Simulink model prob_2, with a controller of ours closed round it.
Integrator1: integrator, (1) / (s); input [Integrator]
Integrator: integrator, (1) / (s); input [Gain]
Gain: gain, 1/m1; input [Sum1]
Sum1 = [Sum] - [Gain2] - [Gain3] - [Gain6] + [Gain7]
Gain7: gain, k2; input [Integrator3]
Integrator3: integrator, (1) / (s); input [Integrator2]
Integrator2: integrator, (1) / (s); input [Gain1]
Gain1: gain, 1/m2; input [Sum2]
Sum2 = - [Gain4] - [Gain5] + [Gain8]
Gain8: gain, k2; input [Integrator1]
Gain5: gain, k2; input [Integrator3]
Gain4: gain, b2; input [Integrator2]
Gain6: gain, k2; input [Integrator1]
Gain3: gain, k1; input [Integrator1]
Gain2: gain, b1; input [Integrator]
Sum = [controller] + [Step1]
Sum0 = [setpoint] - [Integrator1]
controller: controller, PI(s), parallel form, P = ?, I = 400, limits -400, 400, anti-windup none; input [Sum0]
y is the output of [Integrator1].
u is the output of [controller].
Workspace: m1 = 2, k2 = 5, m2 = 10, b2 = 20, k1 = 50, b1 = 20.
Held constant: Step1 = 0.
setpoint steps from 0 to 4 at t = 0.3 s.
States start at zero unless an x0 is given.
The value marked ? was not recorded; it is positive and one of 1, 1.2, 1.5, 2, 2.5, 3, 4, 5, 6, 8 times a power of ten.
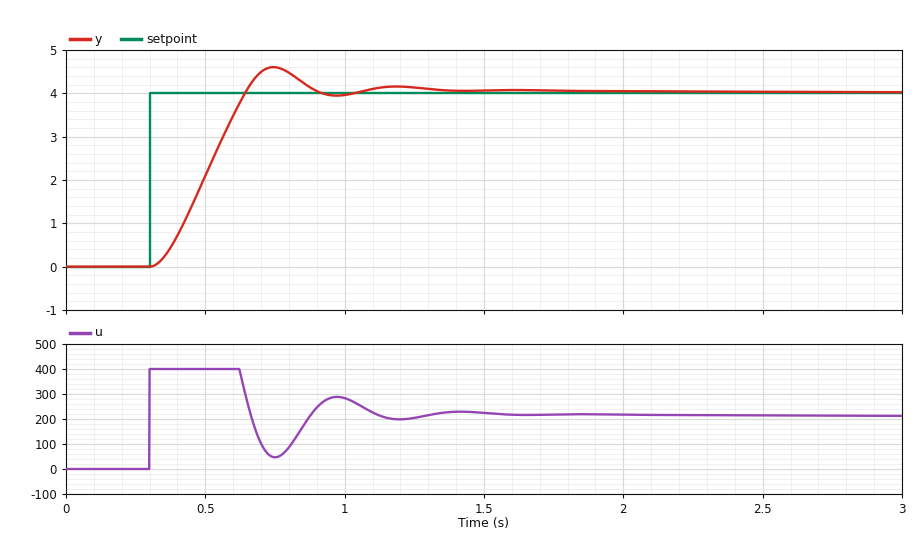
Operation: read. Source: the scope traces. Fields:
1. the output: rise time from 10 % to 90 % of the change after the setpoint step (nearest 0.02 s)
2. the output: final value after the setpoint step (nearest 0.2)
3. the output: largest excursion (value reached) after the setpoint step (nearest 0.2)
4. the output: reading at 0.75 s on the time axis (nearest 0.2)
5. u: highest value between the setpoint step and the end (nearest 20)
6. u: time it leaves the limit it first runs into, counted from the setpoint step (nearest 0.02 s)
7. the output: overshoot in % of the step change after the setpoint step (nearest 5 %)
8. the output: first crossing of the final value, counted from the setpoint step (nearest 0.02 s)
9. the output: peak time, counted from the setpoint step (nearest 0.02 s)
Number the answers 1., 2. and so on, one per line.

1. 0.24 s
2. 4.0
3. 4.6
4. 4.6
5. 400
6. 0.32 s
7. 15 %
8. 0.34 s
9. 0.44 s
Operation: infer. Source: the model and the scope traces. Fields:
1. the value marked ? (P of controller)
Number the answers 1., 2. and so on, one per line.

1. 400
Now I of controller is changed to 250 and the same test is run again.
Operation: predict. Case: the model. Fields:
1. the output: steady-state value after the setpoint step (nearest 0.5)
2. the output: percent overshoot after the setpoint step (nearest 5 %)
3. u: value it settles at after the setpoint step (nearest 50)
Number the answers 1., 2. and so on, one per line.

1. 4.0
2. 10 %
3. 200
